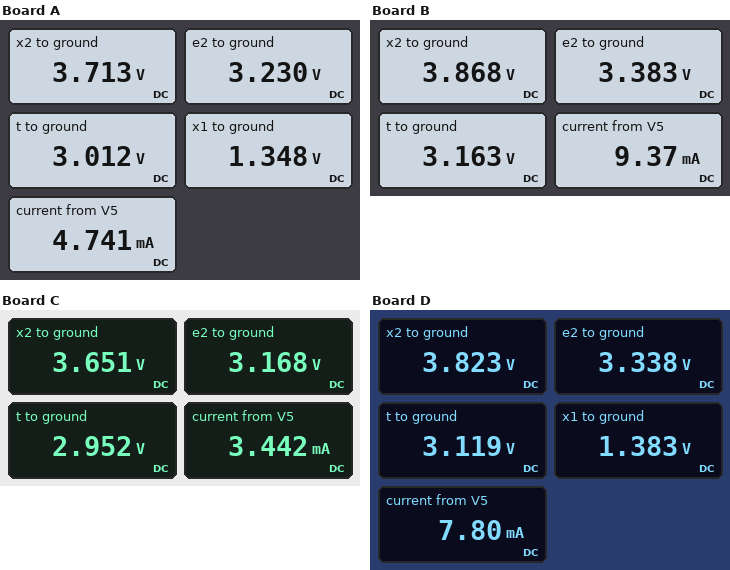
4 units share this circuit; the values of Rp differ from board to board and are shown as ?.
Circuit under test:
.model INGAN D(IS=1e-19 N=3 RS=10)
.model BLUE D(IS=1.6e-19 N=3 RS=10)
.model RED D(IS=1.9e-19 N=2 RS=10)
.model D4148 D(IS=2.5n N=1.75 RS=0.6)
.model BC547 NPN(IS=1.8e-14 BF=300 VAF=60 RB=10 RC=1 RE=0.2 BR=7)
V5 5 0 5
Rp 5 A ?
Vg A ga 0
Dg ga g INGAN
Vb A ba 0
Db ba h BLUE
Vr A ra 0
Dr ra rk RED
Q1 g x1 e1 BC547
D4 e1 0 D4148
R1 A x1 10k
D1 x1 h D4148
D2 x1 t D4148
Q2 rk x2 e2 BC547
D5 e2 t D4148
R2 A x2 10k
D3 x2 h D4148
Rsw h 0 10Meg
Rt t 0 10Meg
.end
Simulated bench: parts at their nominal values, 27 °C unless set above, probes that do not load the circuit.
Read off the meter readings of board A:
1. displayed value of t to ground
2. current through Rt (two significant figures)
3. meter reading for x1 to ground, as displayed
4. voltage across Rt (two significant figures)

3.012 V
300 nA
1.348 V
3.0 V
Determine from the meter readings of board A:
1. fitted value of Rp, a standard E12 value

270 Ω
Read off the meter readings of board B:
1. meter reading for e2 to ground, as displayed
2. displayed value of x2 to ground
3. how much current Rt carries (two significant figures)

3.383 V
3.868 V
320 nA
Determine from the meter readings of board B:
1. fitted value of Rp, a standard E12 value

120 Ω
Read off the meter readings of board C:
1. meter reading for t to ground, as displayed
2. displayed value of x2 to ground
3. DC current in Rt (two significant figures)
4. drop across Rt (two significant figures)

2.952 V
3.651 V
300 nA
3.0 V
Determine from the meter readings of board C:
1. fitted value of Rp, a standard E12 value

390 Ω
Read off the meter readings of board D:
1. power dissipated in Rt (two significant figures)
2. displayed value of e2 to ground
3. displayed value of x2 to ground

970 nW
3.338 V
3.823 V
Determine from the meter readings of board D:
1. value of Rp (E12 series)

150 Ω
